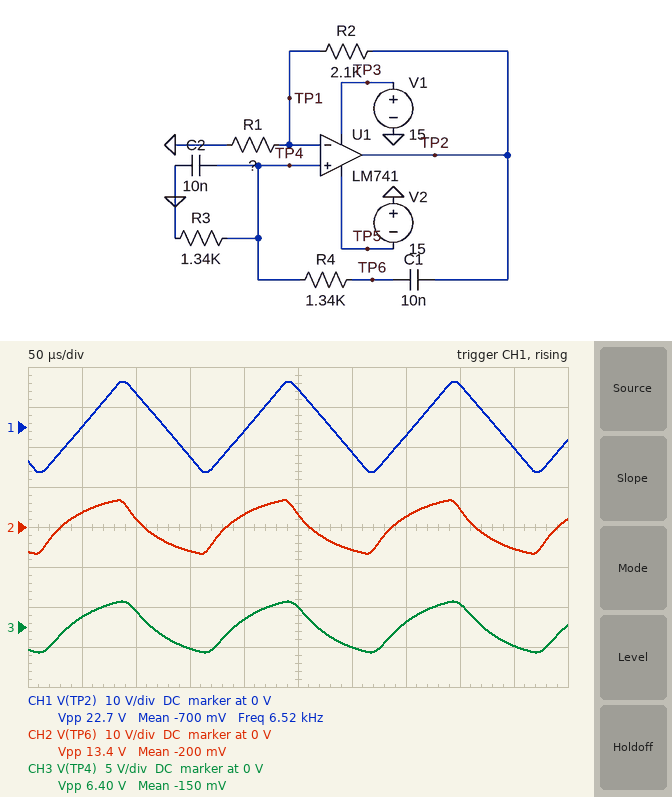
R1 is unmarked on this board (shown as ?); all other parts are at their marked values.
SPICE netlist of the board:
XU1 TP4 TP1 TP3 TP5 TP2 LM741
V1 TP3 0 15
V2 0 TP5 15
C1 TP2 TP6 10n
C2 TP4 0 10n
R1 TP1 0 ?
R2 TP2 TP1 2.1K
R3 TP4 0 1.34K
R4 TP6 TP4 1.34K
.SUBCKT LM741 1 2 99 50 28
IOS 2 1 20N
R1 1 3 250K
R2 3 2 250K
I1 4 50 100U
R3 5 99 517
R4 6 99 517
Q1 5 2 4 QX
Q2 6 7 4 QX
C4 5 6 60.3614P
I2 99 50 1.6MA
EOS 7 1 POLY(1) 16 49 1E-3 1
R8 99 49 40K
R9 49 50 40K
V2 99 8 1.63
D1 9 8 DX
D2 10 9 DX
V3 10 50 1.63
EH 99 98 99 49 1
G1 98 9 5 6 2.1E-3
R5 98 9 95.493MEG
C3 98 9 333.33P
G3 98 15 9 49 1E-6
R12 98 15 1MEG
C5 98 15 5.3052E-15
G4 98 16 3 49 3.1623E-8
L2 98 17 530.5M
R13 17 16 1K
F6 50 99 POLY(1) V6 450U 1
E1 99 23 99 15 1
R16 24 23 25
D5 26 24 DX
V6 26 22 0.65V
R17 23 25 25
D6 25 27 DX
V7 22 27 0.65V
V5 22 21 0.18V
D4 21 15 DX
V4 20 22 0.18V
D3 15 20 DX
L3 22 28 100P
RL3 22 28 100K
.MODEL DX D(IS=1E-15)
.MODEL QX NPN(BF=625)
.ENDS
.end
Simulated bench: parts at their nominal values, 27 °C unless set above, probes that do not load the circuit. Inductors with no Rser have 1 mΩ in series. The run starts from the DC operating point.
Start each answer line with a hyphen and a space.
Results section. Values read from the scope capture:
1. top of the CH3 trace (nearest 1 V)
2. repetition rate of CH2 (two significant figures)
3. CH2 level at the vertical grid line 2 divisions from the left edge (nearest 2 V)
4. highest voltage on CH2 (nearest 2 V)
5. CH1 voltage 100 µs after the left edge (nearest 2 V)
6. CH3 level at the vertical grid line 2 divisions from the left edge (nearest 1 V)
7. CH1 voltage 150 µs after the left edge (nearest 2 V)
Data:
- 3 V
- 6.5 kHz
- 2 V
- 6 V
- 8 V
- 2 V
- -8 V
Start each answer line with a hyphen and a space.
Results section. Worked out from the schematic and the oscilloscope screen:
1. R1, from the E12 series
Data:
- 820 Ω
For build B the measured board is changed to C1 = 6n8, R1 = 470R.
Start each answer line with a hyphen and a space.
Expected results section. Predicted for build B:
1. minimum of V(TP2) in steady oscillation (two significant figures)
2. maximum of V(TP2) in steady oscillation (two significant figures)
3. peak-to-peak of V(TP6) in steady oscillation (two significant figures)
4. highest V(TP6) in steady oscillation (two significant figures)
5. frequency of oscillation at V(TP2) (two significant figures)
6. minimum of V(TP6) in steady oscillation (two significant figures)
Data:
- -14 V
- 14 V
- 11 V
- 5.4 V
- 5.4 kHz
- -5.4 V
